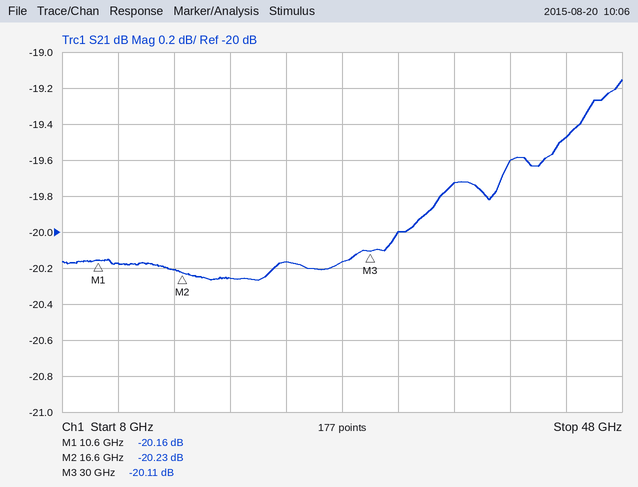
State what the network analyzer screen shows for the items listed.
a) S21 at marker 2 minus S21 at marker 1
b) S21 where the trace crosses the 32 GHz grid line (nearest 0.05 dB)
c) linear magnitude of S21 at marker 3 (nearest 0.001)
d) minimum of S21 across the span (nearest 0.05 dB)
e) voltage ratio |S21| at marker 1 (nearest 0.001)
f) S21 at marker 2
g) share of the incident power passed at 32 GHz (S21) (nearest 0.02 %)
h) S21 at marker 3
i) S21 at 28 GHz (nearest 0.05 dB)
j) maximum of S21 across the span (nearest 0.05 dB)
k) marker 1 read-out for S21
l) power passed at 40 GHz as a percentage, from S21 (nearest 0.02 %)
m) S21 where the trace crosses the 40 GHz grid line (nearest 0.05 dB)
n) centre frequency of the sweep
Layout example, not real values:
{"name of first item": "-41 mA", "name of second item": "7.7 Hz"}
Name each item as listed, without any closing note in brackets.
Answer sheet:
{"S21 at marker 2 minus S21 at marker 1": "-0.07 dB", "S21 where the trace crosses the 32 GHz grid line": "-20.00 dB", "linear magnitude of S21 at marker 3": "0.099", "minimum of S21 across the span": "-20.25 dB", "voltage ratio |S21| at marker 1": "0.098", "S21 at marker 2": "-20.23 dB", "share of the incident power passed at 32 GHz (S21)": "1.00 %", "S21 at marker 3": "-20.11 dB", "S21 at 28 GHz": "-20.15 dB", "maximum of S21 across the span": "-19.15 dB", "marker 1 read-out for S21": "-20.16 dB", "power passed at 40 GHz as a percentage, from S21": "1.10 %", "S21 where the trace crosses the 40 GHz grid line": "-19.60 dB", "centre frequency of the sweep": "28 GHz"}
